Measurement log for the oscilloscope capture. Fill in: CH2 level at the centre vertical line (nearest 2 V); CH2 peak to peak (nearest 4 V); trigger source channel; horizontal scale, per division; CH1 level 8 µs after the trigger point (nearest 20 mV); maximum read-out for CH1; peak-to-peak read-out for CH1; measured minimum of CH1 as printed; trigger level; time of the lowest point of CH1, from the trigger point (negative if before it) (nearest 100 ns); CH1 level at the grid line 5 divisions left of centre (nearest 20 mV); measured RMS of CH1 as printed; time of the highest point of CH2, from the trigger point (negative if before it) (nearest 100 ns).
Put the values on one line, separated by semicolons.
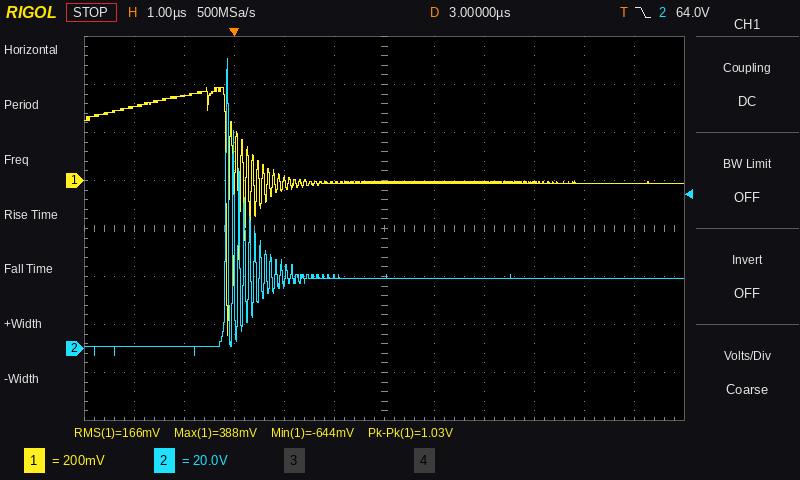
30 V; 124 V; CH2; 1 µs; -20 mV; 388 mV; 1.03 V; -644 mV; 64.0 V; -100 ns; 300 mV; 166 mV; -100 ns
